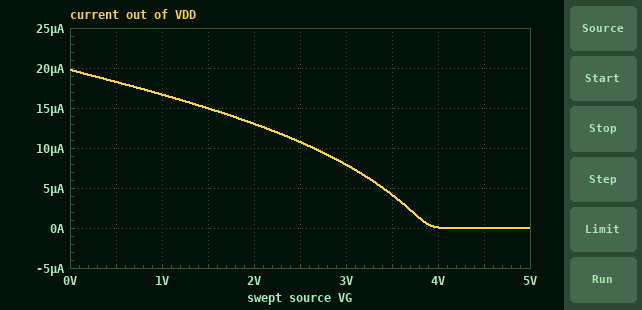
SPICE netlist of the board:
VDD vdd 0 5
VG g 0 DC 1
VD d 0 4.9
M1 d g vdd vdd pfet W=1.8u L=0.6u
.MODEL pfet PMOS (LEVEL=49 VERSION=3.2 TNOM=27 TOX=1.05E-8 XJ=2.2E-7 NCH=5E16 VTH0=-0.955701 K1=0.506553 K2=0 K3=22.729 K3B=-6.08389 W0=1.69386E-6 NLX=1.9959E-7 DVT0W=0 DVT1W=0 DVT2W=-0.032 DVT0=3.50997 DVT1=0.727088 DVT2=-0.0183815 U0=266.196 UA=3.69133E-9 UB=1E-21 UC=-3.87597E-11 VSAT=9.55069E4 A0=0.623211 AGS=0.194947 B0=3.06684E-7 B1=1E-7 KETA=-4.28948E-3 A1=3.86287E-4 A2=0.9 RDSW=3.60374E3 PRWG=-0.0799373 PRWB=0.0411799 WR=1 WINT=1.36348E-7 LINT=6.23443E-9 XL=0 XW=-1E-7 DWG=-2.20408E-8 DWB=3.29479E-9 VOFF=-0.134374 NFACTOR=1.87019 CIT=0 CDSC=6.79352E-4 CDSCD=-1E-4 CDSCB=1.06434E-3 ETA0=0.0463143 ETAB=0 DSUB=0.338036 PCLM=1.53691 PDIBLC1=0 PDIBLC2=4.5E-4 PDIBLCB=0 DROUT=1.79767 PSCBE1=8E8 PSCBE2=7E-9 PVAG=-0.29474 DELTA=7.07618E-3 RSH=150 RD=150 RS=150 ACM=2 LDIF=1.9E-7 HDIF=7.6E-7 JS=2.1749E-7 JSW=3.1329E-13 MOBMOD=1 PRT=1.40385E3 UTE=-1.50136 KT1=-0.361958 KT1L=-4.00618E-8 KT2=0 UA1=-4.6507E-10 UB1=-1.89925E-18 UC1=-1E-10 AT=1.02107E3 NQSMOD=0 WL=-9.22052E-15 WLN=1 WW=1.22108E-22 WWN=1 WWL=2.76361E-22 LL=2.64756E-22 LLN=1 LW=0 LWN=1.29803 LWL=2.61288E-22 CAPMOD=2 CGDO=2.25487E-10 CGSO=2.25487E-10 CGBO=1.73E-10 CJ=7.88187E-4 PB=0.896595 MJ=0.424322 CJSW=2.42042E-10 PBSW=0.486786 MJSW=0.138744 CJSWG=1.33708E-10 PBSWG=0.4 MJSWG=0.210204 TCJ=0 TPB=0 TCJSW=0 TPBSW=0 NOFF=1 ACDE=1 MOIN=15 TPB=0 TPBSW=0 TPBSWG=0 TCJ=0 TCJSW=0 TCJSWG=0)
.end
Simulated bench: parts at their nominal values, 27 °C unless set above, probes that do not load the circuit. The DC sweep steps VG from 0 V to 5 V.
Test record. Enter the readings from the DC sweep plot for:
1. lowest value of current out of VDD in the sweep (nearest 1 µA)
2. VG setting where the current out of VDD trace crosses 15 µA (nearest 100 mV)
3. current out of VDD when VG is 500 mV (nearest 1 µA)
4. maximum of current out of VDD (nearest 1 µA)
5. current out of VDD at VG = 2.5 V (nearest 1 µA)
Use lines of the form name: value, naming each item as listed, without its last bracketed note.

lowest value of current out of VDD in the sweep: 0 A
VG setting where the current out of VDD trace crosses 15 µA: 1.5 V
current out of VDD when VG is 500 mV: 18 µA
maximum of current out of VDD: 20 µA
current out of VDD at VG = 2.5 V: 11 µA
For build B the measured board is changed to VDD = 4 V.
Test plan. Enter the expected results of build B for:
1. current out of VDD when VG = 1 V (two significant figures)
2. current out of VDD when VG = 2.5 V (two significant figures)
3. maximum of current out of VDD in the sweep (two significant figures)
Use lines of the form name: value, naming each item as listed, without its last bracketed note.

current out of VDD when VG = 1 V: -600 µA
current out of VDD when VG = 2.5 V: -580 µA
maximum of current out of VDD in the sweep: -550 µA
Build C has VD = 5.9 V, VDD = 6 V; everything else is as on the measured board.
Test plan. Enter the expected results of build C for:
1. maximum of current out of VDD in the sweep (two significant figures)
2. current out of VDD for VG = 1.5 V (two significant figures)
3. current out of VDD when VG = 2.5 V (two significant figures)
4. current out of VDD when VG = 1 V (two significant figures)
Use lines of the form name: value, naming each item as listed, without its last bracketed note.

maximum of current out of VDD in the sweep: 23 µA
current out of VDD for VG = 1.5 V: 18 µA
current out of VDD when VG = 2.5 V: 15 µA
current out of VDD when VG = 1 V: 20 µA
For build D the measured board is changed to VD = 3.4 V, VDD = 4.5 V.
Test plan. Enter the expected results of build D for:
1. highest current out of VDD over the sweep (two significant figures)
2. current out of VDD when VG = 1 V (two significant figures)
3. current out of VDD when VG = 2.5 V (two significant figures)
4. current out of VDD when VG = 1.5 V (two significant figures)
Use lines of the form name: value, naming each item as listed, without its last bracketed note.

highest current out of VDD over the sweep: 170 µA
current out of VDD when VG = 1 V: 130 µA
current out of VDD when VG = 2.5 V: 40 µA
current out of VDD when VG = 1.5 V: 100 µA
